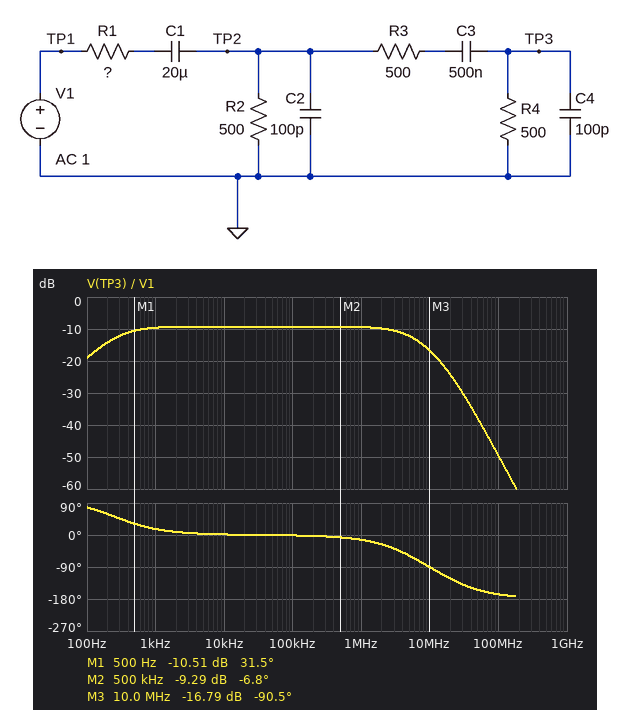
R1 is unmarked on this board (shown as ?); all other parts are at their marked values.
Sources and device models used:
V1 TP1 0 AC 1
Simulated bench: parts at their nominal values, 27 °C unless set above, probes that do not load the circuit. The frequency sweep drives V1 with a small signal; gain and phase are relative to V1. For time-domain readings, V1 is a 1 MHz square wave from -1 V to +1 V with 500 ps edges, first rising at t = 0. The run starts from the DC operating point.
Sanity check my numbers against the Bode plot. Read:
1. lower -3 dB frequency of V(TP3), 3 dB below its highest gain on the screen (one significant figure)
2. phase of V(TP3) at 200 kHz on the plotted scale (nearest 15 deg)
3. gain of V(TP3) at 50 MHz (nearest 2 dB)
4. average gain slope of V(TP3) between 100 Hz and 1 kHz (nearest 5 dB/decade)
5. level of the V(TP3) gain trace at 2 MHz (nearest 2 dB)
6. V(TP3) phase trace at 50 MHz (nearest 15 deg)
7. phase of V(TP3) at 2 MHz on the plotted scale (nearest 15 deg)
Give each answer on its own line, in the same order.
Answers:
300 Hz
0 deg
-38 dB
10 dB/decade
-10 dB
-150 deg
-30 deg
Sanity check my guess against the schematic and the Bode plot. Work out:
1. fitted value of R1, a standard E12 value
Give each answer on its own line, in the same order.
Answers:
150 Ω
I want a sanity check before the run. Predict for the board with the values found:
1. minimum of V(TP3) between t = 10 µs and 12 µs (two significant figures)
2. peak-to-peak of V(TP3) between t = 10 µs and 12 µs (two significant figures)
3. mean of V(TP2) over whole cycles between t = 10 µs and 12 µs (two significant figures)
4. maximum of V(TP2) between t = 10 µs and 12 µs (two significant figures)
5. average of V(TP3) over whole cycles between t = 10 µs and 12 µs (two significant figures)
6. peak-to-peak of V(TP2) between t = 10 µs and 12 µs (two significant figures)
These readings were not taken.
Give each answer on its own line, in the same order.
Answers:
-7.8 mV
690 mV
690 mV
1.4 V
340 mV
1.4 V
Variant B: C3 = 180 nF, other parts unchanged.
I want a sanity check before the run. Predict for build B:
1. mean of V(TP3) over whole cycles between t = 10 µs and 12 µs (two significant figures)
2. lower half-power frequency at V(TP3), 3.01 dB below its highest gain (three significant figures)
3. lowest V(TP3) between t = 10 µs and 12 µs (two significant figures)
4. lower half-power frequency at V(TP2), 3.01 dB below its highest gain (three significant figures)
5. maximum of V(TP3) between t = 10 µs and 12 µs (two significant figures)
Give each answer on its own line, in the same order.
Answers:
330 mV
797 Hz
-20 mV
12.0 Hz
670 mV
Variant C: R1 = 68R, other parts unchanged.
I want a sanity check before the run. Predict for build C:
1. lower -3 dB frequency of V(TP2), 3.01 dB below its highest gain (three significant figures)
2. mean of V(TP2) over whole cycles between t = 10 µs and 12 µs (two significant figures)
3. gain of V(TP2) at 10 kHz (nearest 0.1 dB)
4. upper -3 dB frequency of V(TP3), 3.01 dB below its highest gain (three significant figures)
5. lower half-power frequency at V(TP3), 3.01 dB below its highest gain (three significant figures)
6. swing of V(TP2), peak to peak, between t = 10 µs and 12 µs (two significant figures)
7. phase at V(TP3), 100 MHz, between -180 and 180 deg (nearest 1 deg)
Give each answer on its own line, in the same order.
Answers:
13.4 Hz
830 mV
-1.6 dB
5.73 MHz
307 Hz
1.7 V
-160 deg
